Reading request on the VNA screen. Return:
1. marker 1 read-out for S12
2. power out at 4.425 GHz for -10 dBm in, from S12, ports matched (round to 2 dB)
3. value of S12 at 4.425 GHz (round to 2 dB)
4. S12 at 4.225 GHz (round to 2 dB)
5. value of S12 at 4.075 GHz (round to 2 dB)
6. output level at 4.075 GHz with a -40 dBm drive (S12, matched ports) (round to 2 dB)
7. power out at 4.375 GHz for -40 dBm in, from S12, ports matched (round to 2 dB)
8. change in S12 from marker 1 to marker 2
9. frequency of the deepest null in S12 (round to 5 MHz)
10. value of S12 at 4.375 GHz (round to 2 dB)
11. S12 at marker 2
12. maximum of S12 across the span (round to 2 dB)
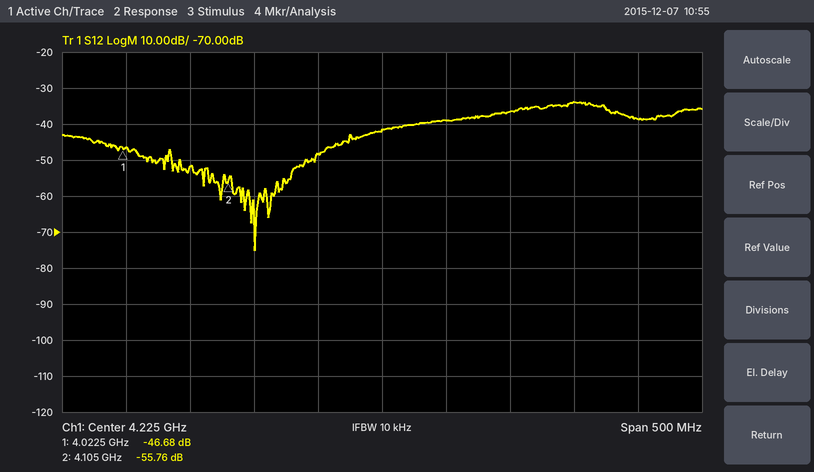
-46.68 dB
-48 dBm
-38 dB
-42 dB
-52 dB
-92 dBm
-74 dBm
-9.08 dB
4.125 GHz
-34 dB
-55.76 dB
-34 dB
